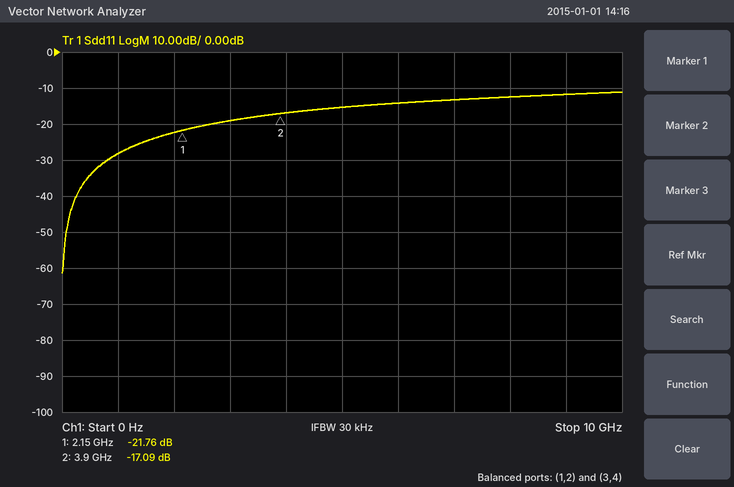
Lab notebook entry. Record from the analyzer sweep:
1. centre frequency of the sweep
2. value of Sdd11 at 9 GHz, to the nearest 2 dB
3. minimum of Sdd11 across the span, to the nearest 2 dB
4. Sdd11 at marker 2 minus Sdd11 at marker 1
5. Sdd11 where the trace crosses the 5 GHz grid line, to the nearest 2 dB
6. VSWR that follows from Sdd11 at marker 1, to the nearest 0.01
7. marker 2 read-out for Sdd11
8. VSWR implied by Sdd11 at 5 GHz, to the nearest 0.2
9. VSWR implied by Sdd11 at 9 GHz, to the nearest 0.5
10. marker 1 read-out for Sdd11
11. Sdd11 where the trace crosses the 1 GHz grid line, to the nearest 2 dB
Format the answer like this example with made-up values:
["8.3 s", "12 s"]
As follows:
["5 GHz", "-12 dB", "-62 dB", "4.67 dB", "-16 dB", "1.18", "-17.09 dB", "1.4", "1.5", "-21.76 dB", "-28 dB"]
